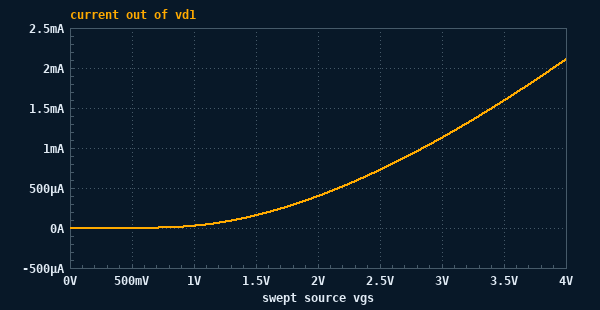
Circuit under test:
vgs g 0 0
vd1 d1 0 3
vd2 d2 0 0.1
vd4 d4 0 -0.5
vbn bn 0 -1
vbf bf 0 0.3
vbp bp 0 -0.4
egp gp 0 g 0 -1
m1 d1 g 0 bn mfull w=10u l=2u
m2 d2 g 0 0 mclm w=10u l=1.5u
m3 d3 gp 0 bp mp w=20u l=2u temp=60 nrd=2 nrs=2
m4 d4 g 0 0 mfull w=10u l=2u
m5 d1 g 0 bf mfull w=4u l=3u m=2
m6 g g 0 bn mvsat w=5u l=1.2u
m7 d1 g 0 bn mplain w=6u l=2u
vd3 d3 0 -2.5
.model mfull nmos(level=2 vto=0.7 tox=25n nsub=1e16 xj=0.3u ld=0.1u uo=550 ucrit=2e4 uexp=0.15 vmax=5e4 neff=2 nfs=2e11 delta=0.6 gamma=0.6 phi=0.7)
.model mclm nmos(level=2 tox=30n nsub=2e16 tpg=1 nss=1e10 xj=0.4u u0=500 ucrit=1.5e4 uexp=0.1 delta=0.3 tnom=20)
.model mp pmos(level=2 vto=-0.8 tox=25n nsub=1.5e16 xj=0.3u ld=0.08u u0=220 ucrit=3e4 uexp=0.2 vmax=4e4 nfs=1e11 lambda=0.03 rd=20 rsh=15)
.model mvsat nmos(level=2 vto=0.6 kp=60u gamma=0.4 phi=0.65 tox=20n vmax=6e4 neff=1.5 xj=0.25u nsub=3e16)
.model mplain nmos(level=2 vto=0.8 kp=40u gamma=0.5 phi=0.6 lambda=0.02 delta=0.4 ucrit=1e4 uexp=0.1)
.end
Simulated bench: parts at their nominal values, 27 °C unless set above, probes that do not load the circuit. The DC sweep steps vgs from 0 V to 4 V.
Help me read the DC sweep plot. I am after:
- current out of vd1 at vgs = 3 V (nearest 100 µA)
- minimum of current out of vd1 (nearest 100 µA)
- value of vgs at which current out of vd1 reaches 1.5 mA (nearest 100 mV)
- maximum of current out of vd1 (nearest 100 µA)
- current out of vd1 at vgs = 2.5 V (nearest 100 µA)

1.1 mA
0 A
3.4 V
2.1 mA
700 µA
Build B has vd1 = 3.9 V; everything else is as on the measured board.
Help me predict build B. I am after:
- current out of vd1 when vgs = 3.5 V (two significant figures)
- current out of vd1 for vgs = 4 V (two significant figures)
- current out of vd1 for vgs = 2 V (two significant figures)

1.7 mA
2.2 mA
420 µA
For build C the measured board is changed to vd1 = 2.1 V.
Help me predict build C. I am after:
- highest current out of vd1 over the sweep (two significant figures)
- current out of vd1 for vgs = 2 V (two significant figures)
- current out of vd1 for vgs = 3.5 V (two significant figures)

2.0 mA
380 µA
1.5 mA
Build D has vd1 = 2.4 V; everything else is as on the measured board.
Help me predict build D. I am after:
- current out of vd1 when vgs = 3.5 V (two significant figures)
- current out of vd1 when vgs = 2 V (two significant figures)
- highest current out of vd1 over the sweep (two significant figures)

1.5 mA
390 µA
2.0 mA
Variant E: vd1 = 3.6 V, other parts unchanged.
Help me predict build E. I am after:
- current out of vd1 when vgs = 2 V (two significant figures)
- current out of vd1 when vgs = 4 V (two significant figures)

410 µA
2.2 mA
